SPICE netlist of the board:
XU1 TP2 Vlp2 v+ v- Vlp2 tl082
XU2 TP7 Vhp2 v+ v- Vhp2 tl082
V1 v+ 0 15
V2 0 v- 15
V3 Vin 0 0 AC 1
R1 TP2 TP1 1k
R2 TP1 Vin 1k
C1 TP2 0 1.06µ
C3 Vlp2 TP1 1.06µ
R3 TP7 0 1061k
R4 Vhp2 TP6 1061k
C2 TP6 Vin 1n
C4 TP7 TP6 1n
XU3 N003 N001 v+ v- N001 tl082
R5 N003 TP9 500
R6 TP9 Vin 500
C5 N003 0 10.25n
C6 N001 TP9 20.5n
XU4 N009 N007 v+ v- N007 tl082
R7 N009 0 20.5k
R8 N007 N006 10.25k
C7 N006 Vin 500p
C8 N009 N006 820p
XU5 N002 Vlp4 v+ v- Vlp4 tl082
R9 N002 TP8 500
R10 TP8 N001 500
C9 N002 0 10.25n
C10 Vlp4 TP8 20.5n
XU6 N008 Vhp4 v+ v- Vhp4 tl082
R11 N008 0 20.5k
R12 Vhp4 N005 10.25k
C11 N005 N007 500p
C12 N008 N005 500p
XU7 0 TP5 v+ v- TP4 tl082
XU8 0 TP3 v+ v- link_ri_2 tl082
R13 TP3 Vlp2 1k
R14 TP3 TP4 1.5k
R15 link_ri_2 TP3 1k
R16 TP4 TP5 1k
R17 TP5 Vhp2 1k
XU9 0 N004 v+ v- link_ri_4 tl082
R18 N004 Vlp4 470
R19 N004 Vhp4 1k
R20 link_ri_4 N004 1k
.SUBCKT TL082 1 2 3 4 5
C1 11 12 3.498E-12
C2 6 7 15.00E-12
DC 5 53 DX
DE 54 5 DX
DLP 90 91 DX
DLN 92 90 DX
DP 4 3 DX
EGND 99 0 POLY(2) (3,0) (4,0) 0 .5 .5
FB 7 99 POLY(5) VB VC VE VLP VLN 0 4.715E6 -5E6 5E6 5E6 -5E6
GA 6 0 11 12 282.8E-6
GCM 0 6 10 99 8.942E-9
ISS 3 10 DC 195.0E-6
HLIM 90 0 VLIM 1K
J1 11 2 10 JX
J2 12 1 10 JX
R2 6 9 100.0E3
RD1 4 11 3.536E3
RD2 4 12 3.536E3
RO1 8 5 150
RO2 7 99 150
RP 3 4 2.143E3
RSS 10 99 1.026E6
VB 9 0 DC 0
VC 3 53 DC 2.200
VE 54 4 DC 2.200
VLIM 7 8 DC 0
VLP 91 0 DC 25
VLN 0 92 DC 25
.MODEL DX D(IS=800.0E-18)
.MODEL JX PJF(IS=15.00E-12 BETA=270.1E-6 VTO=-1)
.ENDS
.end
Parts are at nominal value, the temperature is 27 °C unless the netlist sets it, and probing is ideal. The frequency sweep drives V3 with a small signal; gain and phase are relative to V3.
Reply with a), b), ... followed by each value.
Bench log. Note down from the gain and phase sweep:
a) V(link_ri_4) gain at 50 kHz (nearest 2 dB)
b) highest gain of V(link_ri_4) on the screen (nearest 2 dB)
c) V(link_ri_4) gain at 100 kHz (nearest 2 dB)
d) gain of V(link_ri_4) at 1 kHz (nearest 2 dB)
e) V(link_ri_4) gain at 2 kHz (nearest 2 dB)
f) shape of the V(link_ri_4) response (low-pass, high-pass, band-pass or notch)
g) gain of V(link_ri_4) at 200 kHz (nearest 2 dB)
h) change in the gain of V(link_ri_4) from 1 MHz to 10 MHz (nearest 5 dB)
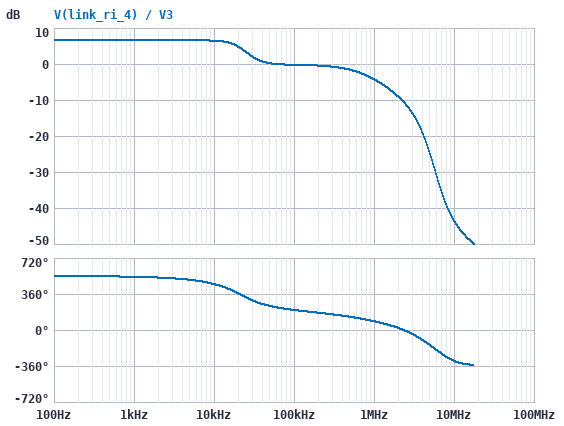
a) 0 dB
b) 6 dB
c) 0 dB
d) 6 dB
e) 6 dB
f) low-pass
g) 0 dB
h) -40 dB
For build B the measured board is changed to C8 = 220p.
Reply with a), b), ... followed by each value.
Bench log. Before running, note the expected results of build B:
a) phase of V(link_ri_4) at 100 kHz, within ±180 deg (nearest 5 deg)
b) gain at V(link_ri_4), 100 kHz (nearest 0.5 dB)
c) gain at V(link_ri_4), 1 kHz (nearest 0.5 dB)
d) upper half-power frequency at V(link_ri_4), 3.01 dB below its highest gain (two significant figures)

a) -145 deg
b) -0.5 dB
c) 6.5 dB
d) 19 kHz
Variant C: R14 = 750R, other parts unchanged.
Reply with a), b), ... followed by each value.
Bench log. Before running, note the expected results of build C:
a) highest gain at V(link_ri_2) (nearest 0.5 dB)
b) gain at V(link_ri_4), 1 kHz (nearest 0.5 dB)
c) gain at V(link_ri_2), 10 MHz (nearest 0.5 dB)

a) 2.5 dB
b) 6.5 dB
c) -40.0 dB
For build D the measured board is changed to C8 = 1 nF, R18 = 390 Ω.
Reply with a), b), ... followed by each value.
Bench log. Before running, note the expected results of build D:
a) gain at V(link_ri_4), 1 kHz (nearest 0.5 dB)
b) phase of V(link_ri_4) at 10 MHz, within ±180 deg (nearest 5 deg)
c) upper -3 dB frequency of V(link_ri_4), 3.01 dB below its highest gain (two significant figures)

a) 8.0 dB
b) 50 deg
c) 22 kHz
